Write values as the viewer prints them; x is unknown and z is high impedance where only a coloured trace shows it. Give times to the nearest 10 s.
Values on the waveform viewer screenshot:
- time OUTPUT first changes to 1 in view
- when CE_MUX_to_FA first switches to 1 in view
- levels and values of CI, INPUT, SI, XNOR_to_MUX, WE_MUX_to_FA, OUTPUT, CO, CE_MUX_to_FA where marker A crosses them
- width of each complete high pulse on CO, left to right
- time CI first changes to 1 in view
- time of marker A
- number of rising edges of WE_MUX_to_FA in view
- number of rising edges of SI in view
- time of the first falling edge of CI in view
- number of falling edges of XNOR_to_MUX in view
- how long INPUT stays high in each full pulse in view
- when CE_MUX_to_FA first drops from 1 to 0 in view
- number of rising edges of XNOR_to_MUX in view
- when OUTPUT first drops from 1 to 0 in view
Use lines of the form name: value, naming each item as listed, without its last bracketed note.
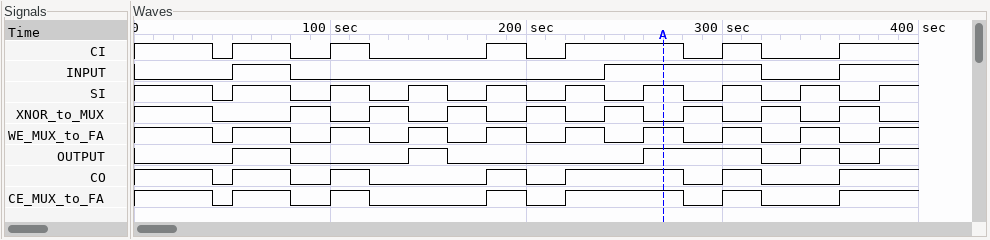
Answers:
time OUTPUT first changes to 1 in view: 50 s
when CE_MUX_to_FA first switches to 1 in view: 50 s
levels and values of CI, INPUT, SI, XNOR_to_MUX, WE_MUX_to_FA, OUTPUT, CO, CE_MUX_to_FA where marker A crosses them: CI=1, INPUT=1, SI=1, XNOR_to_MUX=0, WE_MUX_to_FA=1, OUTPUT=1, CO=1, CE_MUX_to_FA=1
width of each complete high pulse on CO, left to right: 30 s, 20 s, 20 s, 60 s, 20 s
time CI first changes to 1 in view: 50 s
time of marker A: 270 s
number of rising edges of WE_MUX_to_FA in view: 9
number of rising edges of SI in view: 9
time of the first falling edge of CI in view: 40 s
number of falling edges of XNOR_to_MUX in view: 9
how long INPUT stays high in each full pulse in view: 30 s, 80 s
when CE_MUX_to_FA first drops from 1 to 0 in view: 40 s
number of rising edges of XNOR_to_MUX in view: 8
when OUTPUT first drops from 1 to 0 in view: 80 s
